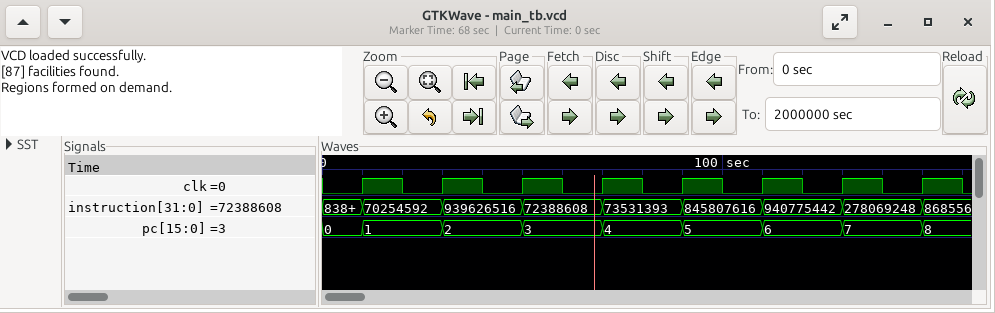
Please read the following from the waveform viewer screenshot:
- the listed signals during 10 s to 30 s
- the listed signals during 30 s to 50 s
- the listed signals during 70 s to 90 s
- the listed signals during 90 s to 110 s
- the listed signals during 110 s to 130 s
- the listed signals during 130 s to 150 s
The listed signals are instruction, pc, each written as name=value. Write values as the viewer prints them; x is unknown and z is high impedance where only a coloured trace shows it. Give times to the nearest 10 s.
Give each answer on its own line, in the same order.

instruction=70254592, pc=1
instruction=939626516, pc=2
instruction=73531393, pc=4
instruction=845807616, pc=5
instruction=940775442, pc=6
instruction=278069248, pc=7
